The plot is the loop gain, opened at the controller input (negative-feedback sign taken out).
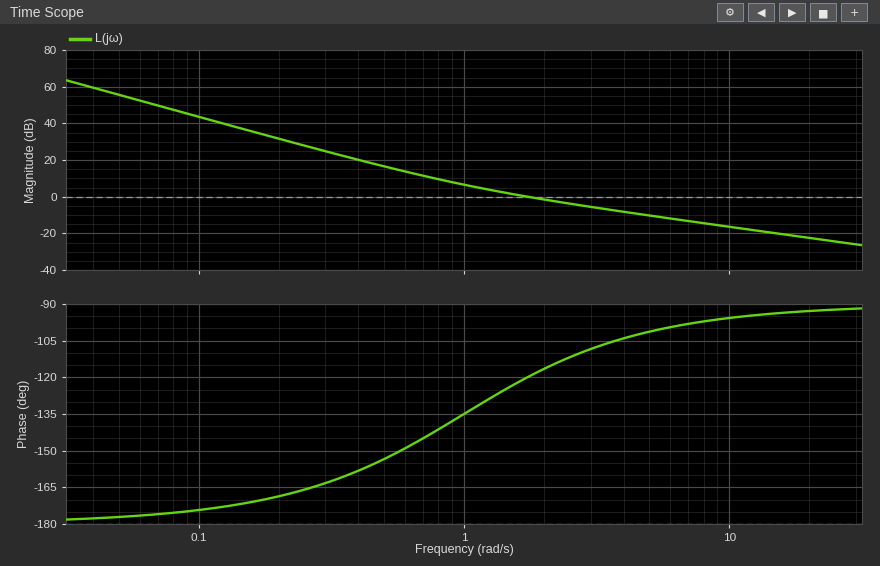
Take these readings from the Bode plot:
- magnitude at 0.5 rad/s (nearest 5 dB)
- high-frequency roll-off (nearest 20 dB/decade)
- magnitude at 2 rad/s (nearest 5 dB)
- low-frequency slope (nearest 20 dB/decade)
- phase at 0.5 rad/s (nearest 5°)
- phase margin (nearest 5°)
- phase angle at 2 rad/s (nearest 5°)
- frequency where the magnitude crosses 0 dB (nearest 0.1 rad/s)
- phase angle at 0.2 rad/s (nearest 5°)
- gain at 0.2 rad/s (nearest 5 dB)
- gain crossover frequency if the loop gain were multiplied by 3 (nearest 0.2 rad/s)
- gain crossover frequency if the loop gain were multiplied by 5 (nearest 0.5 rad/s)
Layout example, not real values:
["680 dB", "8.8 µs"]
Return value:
["15 dB", "-20 dB/decade", "0 dB", "-40 dB/decade", "-155°", "60°", "-115°", "1.7 rad/s", "-170°", "30 dB", "4.6 rad/s", "7.5 rad/s"]
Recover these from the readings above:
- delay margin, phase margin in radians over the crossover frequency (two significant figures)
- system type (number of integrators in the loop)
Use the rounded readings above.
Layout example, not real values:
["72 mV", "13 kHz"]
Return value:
["0.62 s", "2"]
